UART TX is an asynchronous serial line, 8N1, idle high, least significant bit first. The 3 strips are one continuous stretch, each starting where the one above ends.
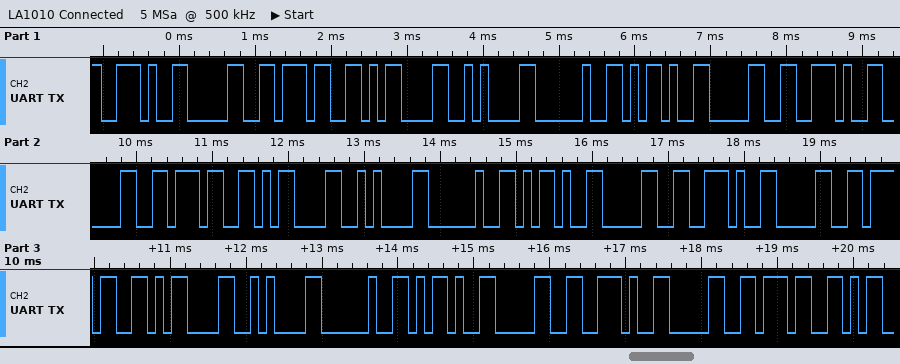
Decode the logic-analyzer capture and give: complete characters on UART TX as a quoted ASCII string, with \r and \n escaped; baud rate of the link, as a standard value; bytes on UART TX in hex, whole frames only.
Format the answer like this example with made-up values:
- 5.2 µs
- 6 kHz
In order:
- ".07\r\n -0.07\r\n -0.07\r\n -0.07"
- 9600 baud
- 0x2E 0x30 0x37 0x0D 0x0A 0x20 0x2D 0x30 0x2E 0x30 0x37 0x0D 0x0A 0x20 0x2D 0x30 0x2E 0x30 0x37 0x0D 0x0A 0x20 0x2D 0x30 0x2E 0x30 0x37
